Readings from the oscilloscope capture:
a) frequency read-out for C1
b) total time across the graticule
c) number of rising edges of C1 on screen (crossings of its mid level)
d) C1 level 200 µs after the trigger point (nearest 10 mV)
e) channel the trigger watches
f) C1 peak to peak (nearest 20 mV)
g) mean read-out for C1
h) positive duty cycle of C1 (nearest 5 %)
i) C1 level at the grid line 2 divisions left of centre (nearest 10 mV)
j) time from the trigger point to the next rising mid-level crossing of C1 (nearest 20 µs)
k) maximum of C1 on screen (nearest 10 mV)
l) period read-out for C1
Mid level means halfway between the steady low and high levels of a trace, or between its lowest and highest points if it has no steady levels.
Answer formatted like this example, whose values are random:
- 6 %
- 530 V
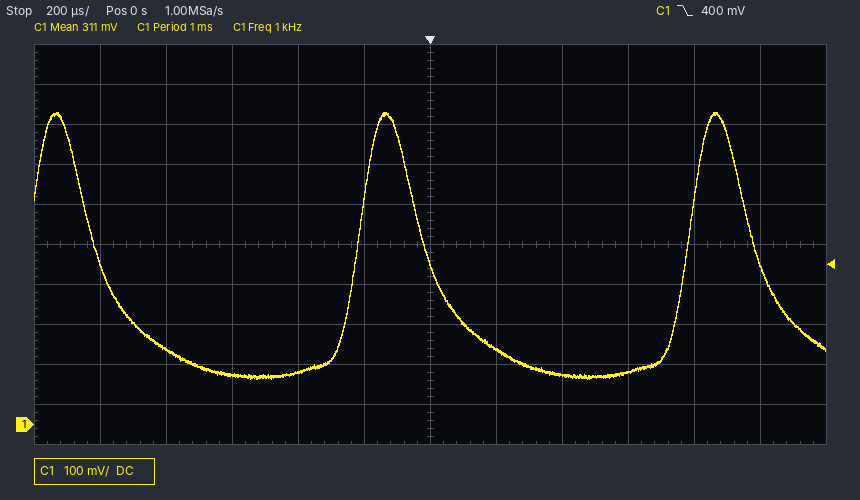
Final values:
- 1 kHz
- 2.4 ms
- 2
- 190 mV
- C1
- 660 mV
- 311 mV
- 20 %
- 130 mV
- 780 µs
- 780 mV
- 1 ms
